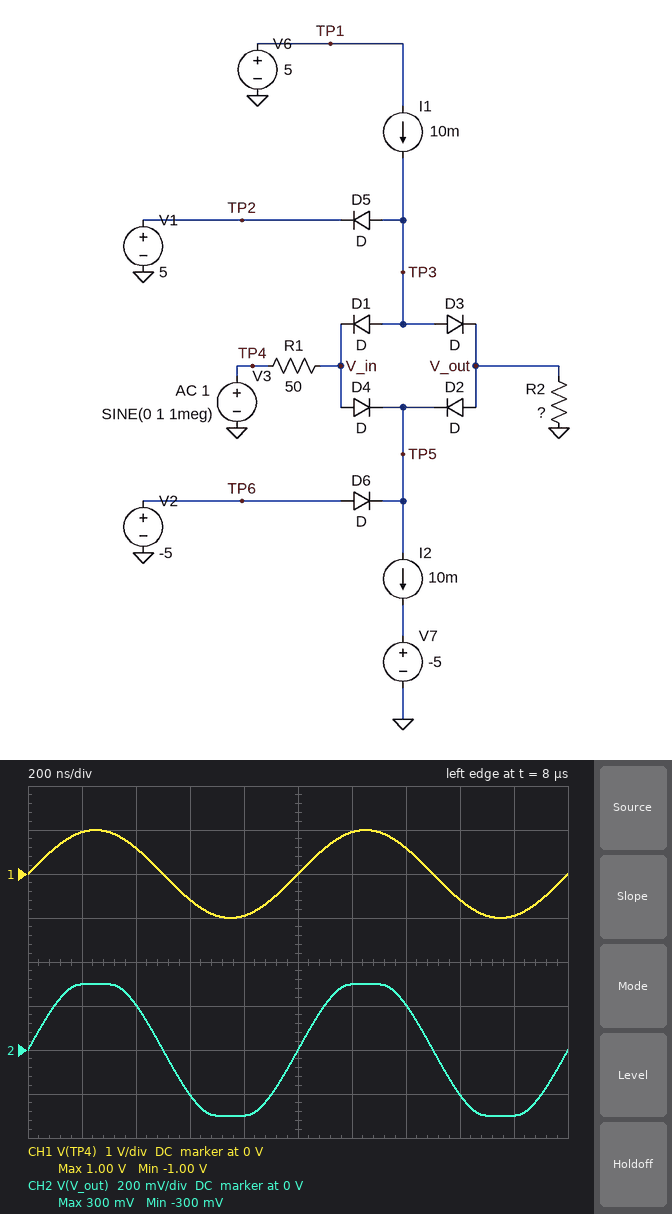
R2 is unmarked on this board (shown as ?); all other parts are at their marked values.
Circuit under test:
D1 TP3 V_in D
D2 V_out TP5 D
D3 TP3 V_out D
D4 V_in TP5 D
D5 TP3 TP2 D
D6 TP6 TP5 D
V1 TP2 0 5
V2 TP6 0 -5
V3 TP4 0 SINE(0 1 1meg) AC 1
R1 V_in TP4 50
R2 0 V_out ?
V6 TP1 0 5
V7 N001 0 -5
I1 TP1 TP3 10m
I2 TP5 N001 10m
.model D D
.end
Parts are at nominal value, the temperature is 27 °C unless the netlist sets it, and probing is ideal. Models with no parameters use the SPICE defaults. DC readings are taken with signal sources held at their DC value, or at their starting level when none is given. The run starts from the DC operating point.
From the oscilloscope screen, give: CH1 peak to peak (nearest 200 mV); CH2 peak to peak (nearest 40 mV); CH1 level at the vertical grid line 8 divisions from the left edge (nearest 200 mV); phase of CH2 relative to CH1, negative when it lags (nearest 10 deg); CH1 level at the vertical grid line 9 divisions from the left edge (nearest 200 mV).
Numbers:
2.0 V
600 mV
-600 mV
0 deg
-1.0 V
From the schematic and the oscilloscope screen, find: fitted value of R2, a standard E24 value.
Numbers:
30 Ω
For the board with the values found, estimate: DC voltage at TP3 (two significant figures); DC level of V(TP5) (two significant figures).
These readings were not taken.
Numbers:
700 mV
-700 mV
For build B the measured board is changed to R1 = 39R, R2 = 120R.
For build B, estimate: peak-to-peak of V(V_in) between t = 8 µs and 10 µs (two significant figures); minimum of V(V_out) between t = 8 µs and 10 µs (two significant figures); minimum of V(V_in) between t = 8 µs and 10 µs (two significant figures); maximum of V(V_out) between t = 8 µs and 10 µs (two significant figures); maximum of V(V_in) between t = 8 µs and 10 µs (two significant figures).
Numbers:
1.5 V
-730 mV
-760 mV
730 mV
760 mV
